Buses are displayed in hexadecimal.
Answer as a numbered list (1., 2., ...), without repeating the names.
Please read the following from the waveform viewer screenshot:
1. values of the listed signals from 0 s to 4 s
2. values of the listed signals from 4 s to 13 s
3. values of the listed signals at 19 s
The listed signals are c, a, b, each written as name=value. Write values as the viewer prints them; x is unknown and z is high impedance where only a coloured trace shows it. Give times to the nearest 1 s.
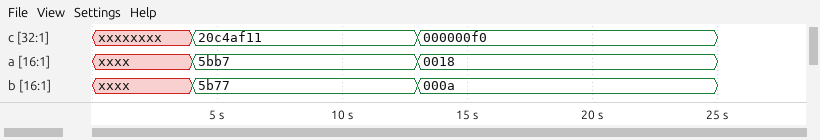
1. c=xxxxxxxx, a=xxxx, b=xxxx
2. c=20c4af11, a=5bb7, b=5b77
3. c=000000f0, a=0018, b=000a
